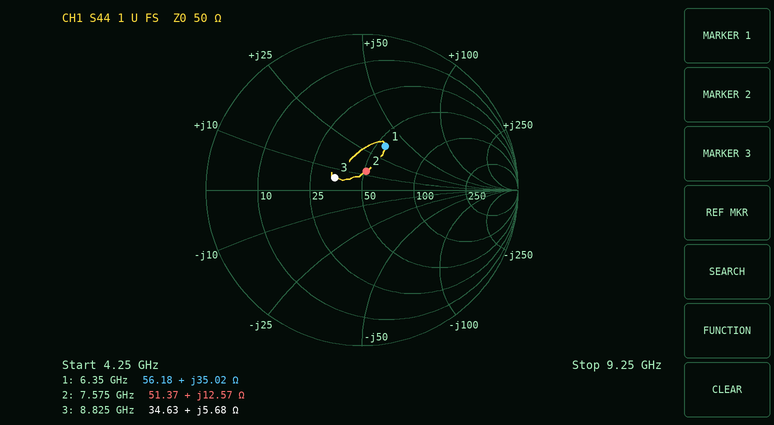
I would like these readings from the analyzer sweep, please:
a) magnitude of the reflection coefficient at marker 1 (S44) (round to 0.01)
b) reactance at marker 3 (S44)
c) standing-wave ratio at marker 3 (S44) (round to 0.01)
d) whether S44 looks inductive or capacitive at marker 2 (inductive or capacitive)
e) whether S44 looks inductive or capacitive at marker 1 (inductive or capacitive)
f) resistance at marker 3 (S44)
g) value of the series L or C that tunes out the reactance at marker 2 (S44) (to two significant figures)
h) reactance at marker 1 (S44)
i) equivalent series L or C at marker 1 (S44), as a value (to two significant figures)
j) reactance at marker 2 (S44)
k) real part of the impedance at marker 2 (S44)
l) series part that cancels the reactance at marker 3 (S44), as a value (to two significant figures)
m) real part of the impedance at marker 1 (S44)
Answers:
0.32
+5.68 Ω
1.48
inductive
inductive
34.63 Ω
1.7 pF
+35.02 Ω
880 pH
+12.57 Ω
51.37 Ω
3.2 pF
56.18 Ω
